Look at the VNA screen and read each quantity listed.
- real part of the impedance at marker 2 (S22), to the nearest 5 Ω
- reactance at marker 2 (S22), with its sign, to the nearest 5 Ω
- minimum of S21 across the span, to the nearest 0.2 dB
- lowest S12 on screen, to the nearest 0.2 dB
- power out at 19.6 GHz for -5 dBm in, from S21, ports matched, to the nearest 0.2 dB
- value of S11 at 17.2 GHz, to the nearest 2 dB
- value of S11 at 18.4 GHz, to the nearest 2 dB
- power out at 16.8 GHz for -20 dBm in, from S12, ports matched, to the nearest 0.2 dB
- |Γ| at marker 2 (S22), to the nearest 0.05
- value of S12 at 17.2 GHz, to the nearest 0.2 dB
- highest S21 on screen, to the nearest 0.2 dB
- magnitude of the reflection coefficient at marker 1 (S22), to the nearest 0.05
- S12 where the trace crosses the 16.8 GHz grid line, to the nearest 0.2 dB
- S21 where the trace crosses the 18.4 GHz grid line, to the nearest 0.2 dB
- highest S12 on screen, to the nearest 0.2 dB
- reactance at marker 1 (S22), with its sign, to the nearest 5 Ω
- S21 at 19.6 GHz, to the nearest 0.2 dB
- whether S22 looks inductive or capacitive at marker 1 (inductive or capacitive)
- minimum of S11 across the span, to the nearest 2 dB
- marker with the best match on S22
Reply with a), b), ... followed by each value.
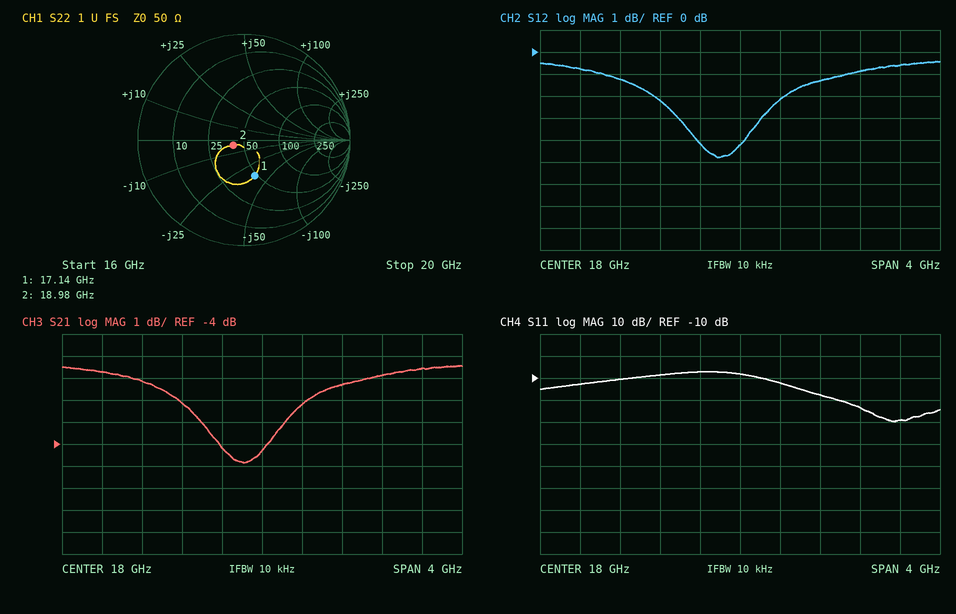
a) 40 Ω
b) -5 Ω
c) -4.8 dB
d) -4.8 dB
e) -5.6 dBm
f) -8 dB
g) -12 dB
h) -21.2 dBm
i) 0.10
j) -2.2 dB
k) -0.4 dB
l) 0.35
m) -1.2 dB
n) -2.2 dB
o) -0.4 dB
p) -35 Ω
q) -0.6 dB
r) capacitive
s) -30 dB
t) marker 2
